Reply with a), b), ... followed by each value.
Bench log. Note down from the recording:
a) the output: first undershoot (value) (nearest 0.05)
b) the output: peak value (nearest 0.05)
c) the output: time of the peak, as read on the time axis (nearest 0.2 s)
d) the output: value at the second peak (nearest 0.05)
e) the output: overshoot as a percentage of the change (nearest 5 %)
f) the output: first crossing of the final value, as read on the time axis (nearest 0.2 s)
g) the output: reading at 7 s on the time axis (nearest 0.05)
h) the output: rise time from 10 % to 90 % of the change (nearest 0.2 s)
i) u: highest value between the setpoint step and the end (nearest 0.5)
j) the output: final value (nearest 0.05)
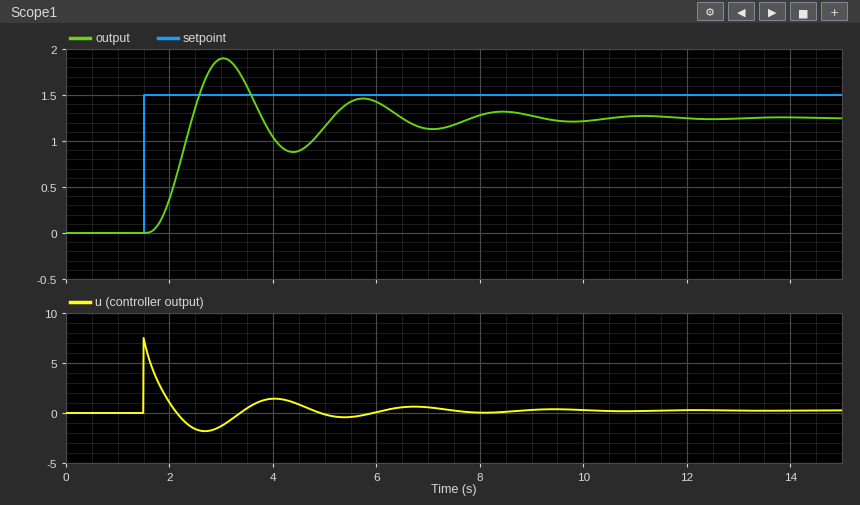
a) 0.90
b) 1.90
c) 3.0 s
d) 1.45
e) 50 %
f) 2.4 s
g) 1.15
h) 0.6 s
i) 7.5
j) 1.25
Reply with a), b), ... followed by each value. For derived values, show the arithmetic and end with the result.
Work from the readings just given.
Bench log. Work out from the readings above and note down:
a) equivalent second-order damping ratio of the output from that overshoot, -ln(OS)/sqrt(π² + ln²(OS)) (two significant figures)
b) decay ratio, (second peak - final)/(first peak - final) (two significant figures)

a) ln(0.5) = -0.693; 0.693 / sqrt(9.870 + 0.480) = 0.22
b) (1.45 - 1.25) / (1.9 - 1.25) = 0.31
